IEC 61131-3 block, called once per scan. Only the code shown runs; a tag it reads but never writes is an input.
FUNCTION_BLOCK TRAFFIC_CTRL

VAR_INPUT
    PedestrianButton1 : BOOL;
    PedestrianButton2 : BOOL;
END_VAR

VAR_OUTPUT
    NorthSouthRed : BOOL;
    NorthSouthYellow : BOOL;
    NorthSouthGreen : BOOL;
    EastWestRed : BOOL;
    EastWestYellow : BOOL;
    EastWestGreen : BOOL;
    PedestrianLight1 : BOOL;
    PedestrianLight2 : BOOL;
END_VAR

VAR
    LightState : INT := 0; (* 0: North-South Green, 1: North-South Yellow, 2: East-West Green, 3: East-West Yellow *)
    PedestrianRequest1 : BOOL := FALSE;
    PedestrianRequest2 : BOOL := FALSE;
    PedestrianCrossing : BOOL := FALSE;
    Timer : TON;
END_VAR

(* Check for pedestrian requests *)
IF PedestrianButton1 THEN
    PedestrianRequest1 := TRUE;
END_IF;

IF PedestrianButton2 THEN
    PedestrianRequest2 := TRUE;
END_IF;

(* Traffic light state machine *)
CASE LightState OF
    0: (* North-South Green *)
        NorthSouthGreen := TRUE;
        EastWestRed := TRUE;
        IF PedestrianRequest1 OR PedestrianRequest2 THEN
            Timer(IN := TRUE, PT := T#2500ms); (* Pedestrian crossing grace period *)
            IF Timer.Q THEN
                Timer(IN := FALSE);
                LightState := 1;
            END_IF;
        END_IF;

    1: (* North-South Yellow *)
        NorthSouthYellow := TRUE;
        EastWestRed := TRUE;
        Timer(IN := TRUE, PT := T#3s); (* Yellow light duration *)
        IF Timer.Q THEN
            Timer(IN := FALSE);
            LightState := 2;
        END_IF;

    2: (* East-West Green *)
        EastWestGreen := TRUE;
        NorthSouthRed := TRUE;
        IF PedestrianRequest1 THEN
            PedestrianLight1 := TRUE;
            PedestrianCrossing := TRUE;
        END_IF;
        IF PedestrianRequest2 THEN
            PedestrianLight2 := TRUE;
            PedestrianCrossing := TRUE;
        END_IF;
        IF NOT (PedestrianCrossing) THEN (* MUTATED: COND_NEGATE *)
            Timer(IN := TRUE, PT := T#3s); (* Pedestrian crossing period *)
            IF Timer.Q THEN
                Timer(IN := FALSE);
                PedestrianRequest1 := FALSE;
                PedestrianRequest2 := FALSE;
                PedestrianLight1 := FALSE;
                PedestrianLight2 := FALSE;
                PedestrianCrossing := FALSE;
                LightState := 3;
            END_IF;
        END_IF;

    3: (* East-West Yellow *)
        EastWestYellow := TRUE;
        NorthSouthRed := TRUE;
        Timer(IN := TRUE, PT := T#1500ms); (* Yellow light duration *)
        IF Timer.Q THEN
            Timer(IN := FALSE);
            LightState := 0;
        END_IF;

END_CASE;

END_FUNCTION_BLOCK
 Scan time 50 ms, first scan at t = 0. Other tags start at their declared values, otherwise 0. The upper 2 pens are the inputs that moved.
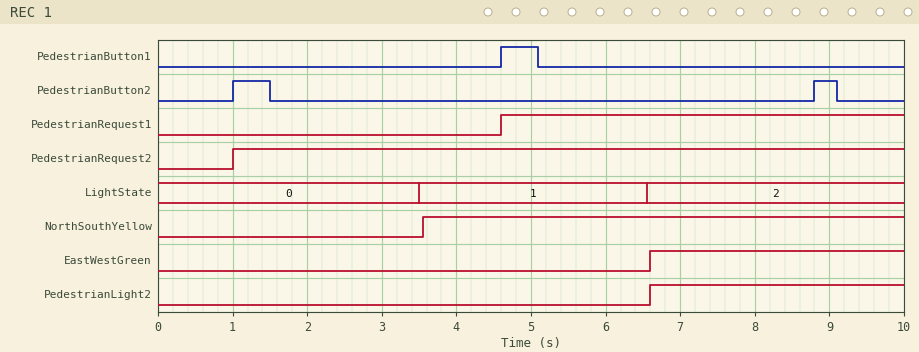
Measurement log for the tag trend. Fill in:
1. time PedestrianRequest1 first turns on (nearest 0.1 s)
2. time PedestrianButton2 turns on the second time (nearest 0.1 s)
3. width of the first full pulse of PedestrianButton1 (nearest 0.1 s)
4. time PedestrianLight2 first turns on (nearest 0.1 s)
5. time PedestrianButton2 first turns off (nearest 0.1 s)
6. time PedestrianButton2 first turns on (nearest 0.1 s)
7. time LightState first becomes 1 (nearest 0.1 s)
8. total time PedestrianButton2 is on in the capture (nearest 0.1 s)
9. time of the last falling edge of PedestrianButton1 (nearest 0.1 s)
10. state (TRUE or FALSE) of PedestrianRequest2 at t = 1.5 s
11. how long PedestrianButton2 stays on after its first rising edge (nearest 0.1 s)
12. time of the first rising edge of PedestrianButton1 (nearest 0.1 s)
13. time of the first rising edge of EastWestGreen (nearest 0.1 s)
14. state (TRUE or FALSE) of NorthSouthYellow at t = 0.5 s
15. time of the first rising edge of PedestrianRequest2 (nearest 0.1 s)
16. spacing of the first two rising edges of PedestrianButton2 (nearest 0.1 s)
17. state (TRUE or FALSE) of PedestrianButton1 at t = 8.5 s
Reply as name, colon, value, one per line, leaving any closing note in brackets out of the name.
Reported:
time PedestrianRequest1 first turns on: 4.6 s
time PedestrianButton2 turns on the second time: 8.8 s
width of the first full pulse of PedestrianButton1: 0.5 s
time PedestrianLight2 first turns on: 6.6 s
time PedestrianButton2 first turns off: 1.5 s
time PedestrianButton2 first turns on: 1.0 s
time LightState first becomes 1: 3.5 s
total time PedestrianButton2 is on in the capture: 0.8 s
time of the last falling edge of PedestrianButton1: 5.1 s
state (TRUE or FALSE) of PedestrianRequest2 at t = 1.5 s: TRUE
how long PedestrianButton2 stays on after its first rising edge: 0.5 s
time of the first rising edge of PedestrianButton1: 4.6 s
time of the first rising edge of EastWestGreen: 6.6 s
state (TRUE or FALSE) of NorthSouthYellow at t = 0.5 s: FALSE
time of the first rising edge of PedestrianRequest2: 1.0 s
spacing of the first two rising edges of PedestrianButton2: 7.8 s
state (TRUE or FALSE) of PedestrianButton1 at t = 8.5 s: FALSE
